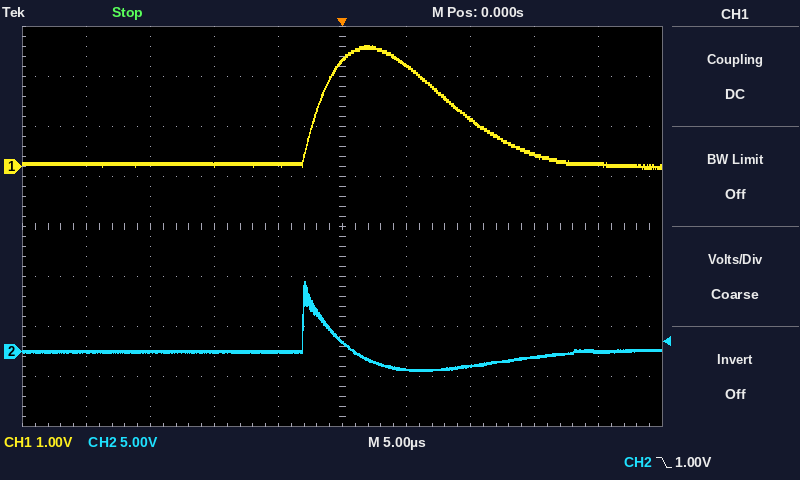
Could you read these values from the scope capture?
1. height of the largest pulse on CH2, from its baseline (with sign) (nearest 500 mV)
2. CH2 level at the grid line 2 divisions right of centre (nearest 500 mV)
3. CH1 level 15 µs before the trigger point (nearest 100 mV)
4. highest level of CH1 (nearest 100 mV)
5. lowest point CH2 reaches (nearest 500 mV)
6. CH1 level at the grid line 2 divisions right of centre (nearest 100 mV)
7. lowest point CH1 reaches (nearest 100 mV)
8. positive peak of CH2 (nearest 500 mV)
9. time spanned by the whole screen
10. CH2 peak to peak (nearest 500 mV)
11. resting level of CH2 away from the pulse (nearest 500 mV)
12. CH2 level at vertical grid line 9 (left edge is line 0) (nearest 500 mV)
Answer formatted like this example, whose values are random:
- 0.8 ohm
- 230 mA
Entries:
- +7.0 V
- -1.5 V
- 100 mV
- 2.4 V
- -2.0 V
- 1.0 V
- 0.0 V
- 7.0 V
- 50 µs
- 9.0 V
- 0.0 V
- 0.0 V
